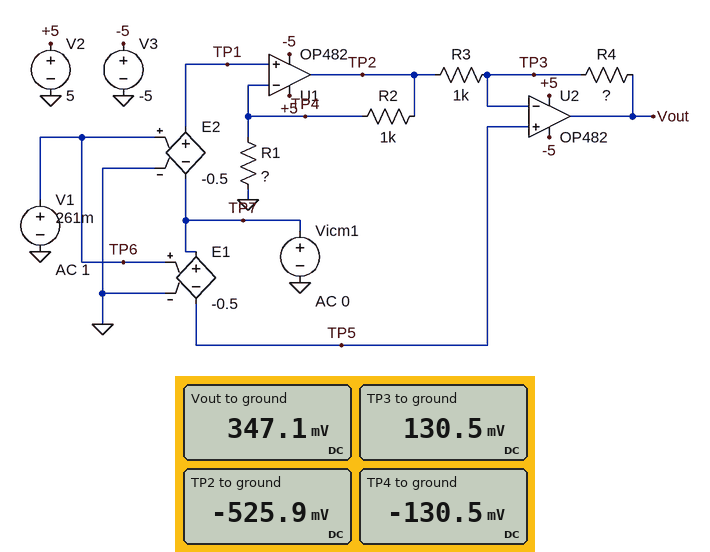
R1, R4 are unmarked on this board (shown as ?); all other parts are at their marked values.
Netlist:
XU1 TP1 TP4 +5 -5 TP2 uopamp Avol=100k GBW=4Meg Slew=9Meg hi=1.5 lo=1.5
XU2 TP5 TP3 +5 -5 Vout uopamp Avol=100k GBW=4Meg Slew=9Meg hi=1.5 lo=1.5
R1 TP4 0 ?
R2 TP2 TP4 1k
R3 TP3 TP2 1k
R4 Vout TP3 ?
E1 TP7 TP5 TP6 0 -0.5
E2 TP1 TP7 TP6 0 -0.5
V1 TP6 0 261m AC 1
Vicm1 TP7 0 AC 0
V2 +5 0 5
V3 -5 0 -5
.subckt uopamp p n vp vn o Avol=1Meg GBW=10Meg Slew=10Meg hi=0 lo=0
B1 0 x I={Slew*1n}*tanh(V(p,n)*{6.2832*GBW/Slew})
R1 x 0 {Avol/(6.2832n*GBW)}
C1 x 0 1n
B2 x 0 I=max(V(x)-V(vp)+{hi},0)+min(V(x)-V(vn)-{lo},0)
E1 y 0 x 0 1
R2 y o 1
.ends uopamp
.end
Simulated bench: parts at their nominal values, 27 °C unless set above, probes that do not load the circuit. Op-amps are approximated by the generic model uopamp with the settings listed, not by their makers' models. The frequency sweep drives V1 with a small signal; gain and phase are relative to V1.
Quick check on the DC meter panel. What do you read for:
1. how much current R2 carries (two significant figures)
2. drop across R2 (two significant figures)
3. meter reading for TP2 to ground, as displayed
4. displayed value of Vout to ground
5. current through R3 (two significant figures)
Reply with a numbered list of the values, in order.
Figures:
1. 400 µA
2. 400 mV
3. -525.9 mV
4. 347.1 mV
5. 660 µA
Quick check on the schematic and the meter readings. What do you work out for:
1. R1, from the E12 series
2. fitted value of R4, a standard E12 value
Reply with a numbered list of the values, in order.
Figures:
1. 330 Ω
2. 330 Ω
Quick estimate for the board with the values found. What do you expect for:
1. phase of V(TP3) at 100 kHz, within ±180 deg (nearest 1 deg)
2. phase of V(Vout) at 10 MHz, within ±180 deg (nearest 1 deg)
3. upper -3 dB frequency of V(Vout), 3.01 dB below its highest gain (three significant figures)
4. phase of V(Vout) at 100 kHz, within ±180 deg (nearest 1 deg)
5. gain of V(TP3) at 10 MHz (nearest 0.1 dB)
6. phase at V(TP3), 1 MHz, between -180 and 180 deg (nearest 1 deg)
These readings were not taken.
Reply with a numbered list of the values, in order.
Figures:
1. -4 deg
2. -79 deg
3. 1.14 MHz
4. -5 deg
5. -20.3 dB
6. -30 deg
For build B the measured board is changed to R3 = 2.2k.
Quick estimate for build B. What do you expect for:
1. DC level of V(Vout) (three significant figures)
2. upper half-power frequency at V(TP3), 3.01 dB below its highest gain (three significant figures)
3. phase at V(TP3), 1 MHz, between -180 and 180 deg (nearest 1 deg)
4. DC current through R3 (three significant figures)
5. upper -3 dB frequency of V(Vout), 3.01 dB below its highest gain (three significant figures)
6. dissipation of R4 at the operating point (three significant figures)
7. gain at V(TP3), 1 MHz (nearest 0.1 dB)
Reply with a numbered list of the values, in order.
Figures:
1. 229 mV
2. 2.51 MHz
3. -21 deg
4. 298 µA
5. 1.53 MHz
6. 29.4 µW
7. -7.0 dB
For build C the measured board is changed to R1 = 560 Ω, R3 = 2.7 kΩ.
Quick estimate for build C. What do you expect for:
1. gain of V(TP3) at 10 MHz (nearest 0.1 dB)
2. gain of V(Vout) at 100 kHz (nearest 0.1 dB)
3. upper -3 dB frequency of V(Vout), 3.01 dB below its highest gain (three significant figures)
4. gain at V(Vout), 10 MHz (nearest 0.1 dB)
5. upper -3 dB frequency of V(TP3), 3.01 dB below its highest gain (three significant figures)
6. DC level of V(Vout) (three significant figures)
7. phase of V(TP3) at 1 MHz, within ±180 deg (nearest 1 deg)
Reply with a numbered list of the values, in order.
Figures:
1. -16.6 dB
2. -2.7 dB
3. 2.28 MHz
4. -14.4 dB
5. 2.84 MHz
6. 191 mV
7. -19 deg
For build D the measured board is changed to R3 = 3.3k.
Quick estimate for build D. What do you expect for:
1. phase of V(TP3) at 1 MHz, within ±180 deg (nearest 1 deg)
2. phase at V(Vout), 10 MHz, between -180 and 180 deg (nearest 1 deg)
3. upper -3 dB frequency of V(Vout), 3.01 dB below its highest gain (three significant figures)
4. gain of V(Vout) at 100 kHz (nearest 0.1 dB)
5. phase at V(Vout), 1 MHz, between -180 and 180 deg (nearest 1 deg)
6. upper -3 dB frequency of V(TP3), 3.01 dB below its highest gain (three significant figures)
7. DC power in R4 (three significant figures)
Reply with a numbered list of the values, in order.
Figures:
1. -18 deg
2. -72 deg
3. 1.89 MHz
4. -2.5 dB
5. -24 deg
6. 2.95 MHz
7. 13.1 µW
